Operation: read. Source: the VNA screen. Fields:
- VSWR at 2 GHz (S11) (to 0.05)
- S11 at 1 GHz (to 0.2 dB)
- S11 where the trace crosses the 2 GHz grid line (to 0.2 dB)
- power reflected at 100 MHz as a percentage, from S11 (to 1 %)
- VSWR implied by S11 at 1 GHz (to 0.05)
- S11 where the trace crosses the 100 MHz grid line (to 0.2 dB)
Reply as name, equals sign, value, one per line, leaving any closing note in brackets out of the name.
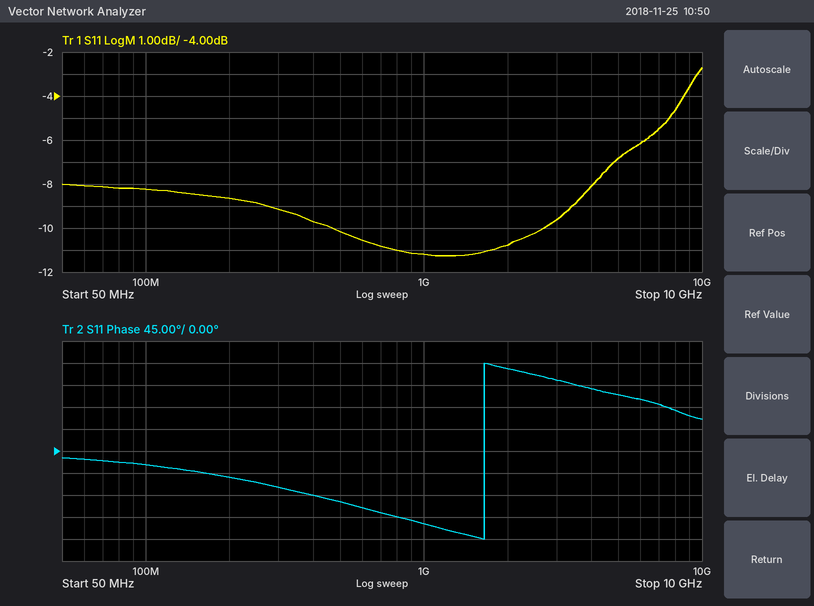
VSWR at 2 GHz (S11) = 1.80
S11 at 1 GHz = -11.2 dB
S11 where the trace crosses the 2 GHz grid line = -10.8 dB
power reflected at 100 MHz as a percentage, from S11 = 15 %
VSWR implied by S11 at 1 GHz = 1.75
S11 where the trace crosses the 100 MHz grid line = -8.2 dB
